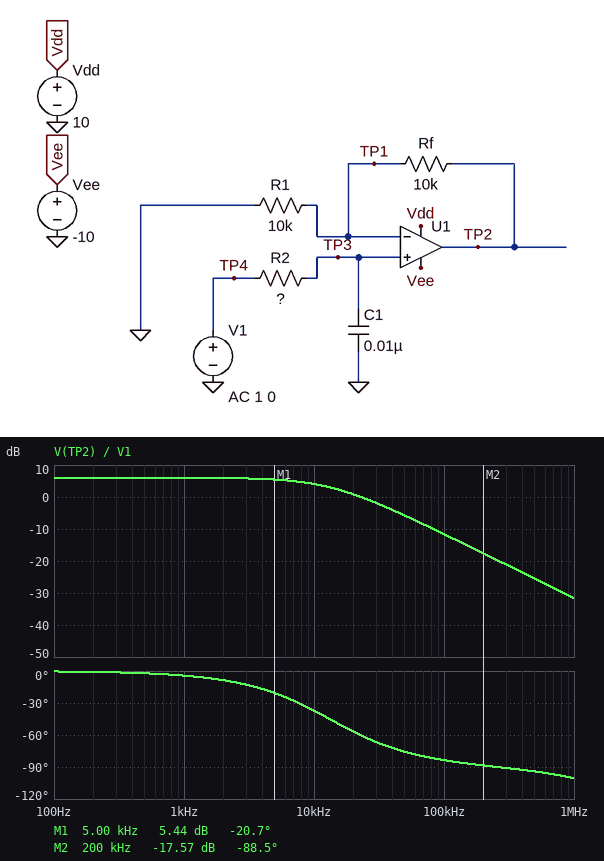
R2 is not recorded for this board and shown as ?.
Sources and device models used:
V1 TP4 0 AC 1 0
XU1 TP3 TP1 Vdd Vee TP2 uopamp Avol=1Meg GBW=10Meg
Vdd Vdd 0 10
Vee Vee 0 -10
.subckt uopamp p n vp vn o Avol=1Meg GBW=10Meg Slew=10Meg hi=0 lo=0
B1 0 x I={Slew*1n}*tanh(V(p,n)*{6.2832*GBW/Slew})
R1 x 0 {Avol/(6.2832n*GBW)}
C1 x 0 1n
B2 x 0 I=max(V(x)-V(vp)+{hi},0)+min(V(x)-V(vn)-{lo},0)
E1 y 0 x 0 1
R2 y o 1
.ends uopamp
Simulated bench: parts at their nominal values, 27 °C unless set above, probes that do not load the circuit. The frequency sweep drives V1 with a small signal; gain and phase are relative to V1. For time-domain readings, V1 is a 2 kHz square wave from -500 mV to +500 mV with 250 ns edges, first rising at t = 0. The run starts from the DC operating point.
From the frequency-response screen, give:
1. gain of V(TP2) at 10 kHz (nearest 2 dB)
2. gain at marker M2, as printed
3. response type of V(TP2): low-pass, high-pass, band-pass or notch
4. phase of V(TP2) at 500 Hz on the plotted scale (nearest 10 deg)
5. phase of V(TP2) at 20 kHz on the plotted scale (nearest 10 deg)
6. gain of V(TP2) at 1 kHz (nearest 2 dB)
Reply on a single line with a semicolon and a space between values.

4 dB; -17.57 dB; low-pass; 0 deg; -60 deg; 6 dB
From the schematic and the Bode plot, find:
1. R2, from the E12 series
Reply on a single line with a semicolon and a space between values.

1.2 kΩ
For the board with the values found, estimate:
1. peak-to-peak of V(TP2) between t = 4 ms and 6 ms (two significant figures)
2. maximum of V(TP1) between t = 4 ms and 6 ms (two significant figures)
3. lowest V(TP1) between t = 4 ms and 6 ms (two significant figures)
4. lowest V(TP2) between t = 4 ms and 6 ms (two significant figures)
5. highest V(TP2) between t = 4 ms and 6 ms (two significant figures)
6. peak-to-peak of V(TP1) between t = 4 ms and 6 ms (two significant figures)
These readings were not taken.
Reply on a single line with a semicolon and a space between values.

2.0 V; 500 mV; -500 mV; -1.0 V; 1.0 V; 1.0 V
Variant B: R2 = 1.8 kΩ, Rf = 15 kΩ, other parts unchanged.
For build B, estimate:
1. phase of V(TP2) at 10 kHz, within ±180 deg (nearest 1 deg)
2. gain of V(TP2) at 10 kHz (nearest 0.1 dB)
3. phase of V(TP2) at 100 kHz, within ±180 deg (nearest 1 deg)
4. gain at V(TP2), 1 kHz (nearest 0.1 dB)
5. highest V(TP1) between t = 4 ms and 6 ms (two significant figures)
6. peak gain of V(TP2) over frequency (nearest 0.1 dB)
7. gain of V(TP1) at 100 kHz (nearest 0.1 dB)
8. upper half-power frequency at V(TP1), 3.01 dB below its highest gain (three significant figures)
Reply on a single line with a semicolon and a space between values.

-49 deg; 4.4 dB; -86 deg; 7.9 dB; 500 mV; 8.0 dB; -21.1 dB; 8.84 kHz
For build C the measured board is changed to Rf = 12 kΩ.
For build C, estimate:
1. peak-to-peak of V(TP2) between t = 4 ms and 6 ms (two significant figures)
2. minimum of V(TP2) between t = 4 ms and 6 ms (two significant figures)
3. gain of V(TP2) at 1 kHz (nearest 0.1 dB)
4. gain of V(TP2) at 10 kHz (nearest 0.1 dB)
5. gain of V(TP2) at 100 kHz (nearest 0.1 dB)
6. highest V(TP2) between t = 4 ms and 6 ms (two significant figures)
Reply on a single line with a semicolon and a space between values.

2.2 V; -1.1 V; 6.8 dB; 4.9 dB; -10.8 dB; 1.1 V
